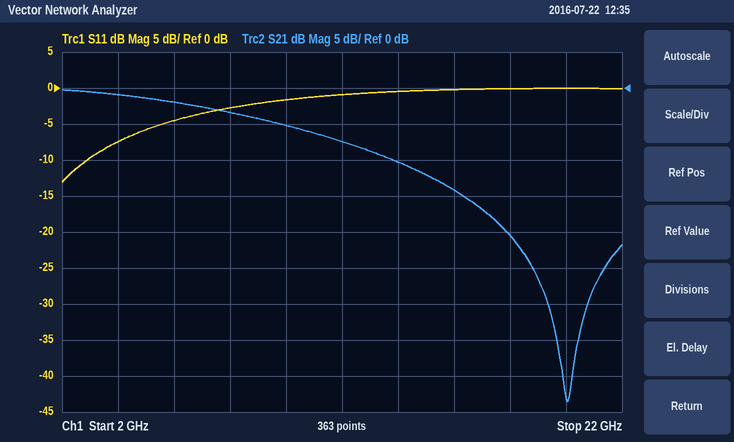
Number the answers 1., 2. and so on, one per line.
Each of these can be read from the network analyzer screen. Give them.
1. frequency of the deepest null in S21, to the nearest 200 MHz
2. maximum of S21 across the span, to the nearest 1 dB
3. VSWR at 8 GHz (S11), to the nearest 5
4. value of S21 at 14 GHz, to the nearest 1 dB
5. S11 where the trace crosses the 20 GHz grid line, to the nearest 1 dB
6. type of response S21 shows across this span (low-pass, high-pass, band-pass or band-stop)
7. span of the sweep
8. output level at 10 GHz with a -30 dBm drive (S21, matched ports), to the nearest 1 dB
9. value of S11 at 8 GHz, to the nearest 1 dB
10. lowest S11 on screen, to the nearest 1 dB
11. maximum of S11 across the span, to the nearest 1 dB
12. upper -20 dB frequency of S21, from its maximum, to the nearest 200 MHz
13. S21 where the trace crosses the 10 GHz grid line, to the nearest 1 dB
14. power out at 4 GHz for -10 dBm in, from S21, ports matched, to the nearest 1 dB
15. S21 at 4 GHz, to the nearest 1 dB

1. 20.0 GHz
2. 0 dB
3. 5
4. -10 dB
5. 0 dB
6. low-pass
7. 20 GHz
8. -35 dBm
9. -3 dB
10. -13 dB
11. 0 dB
12. 18.0 GHz
13. -5 dB
14. -11 dBm
15. -1 dB
